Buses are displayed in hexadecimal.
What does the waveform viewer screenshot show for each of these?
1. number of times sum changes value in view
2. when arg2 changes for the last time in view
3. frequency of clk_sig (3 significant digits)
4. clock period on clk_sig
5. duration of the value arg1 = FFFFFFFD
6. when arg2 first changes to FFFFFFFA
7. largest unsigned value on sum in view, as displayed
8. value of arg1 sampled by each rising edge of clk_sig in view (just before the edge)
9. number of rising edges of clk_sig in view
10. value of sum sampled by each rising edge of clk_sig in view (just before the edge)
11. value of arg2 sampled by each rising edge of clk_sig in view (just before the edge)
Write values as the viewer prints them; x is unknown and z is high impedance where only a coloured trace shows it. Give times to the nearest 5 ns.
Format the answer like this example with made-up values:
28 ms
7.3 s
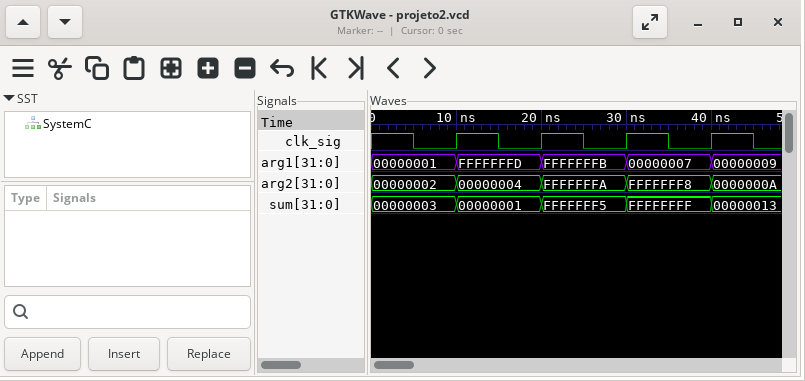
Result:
4
40 ns
100 MHz
10 ns
10 ns
20 ns
FFFFFFFF
00000001, FFFFFFFD, FFFFFFFB, 00000007
4
00000003, 00000001, FFFFFFF5, FFFFFFFF
00000002, 00000004, FFFFFFFA, FFFFFFF8
